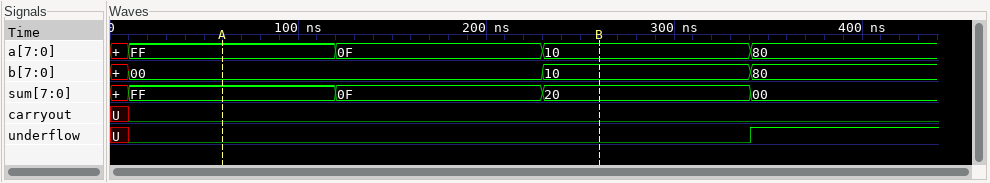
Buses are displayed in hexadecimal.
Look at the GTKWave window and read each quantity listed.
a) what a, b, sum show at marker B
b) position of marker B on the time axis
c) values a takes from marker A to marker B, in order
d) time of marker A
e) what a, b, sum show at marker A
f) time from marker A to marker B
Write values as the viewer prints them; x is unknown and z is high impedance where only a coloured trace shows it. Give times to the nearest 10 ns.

a=10, b=10, sum=20
260 ns
FF, 0F, 10
60 ns
a=FF, b=00, sum=FF
200 ns
